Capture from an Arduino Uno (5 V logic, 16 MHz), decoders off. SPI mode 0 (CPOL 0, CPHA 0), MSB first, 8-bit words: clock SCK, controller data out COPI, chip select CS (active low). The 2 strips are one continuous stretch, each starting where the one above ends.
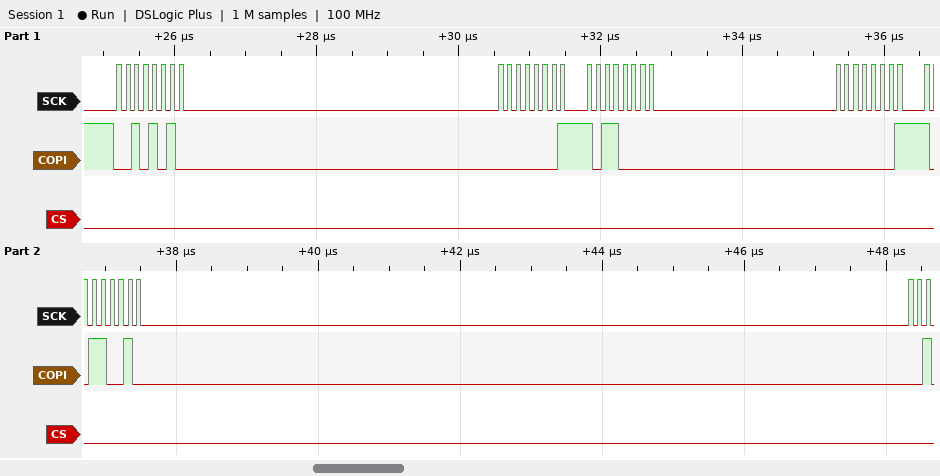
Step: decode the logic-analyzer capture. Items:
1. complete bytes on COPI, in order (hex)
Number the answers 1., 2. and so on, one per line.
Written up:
1. 0x2A 0x01 0xB0 0x01 0xB2
